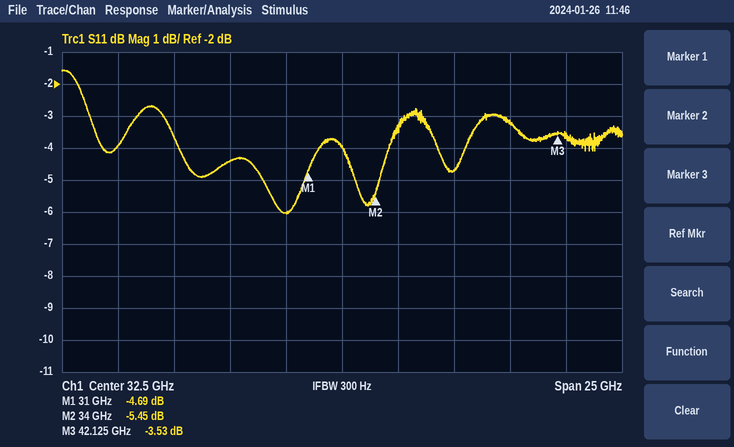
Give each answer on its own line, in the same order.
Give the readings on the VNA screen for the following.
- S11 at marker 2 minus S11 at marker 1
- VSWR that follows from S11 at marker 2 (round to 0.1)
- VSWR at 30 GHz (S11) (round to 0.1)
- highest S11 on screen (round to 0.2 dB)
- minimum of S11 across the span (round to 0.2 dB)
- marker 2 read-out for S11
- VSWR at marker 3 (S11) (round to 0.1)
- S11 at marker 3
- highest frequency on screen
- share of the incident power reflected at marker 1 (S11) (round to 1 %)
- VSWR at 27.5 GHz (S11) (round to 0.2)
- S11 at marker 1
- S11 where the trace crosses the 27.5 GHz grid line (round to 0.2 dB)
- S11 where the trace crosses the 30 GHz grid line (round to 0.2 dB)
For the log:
-0.76 dB
3.3
3.0
-1.6 dB
-6.0 dB
-5.45 dB
5.0
-3.53 dB
45 GHz
34 %
4.0
-4.69 dB
-4.4 dB
-6.0 dB
